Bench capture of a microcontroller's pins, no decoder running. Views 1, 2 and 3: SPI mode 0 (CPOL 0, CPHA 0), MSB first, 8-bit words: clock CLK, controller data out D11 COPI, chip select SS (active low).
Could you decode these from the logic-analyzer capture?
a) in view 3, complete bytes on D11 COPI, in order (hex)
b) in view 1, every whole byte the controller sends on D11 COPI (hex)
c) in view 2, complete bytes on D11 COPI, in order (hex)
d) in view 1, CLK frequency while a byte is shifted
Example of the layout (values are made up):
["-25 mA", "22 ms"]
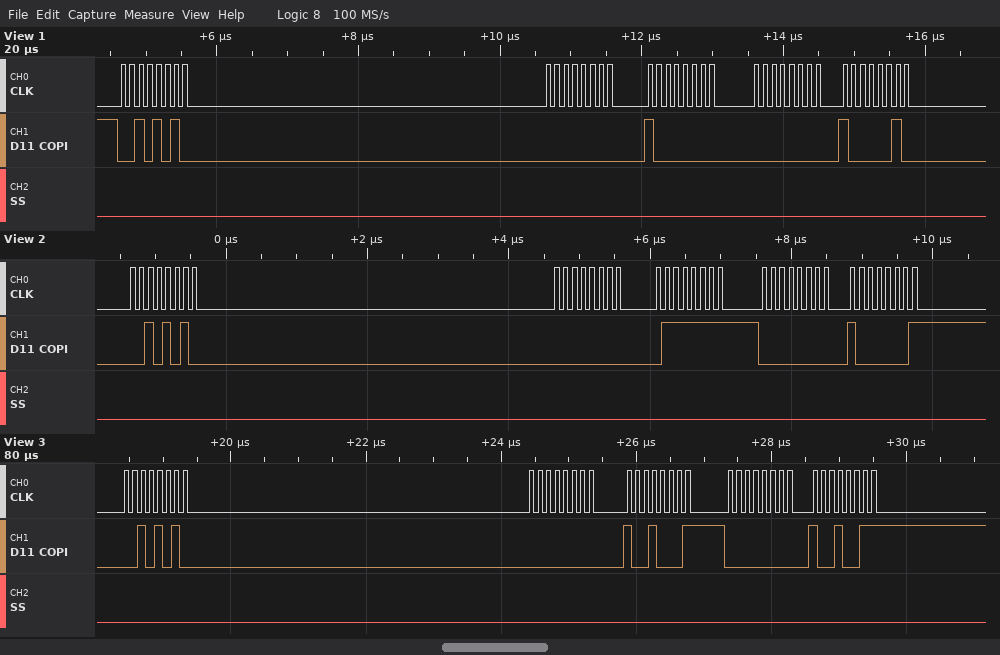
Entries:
["0x2A 0x00 0x91 0x00 0x93", "2A 00 80 00 82", "2A 00 7F 00 81", "8 MHz"]
